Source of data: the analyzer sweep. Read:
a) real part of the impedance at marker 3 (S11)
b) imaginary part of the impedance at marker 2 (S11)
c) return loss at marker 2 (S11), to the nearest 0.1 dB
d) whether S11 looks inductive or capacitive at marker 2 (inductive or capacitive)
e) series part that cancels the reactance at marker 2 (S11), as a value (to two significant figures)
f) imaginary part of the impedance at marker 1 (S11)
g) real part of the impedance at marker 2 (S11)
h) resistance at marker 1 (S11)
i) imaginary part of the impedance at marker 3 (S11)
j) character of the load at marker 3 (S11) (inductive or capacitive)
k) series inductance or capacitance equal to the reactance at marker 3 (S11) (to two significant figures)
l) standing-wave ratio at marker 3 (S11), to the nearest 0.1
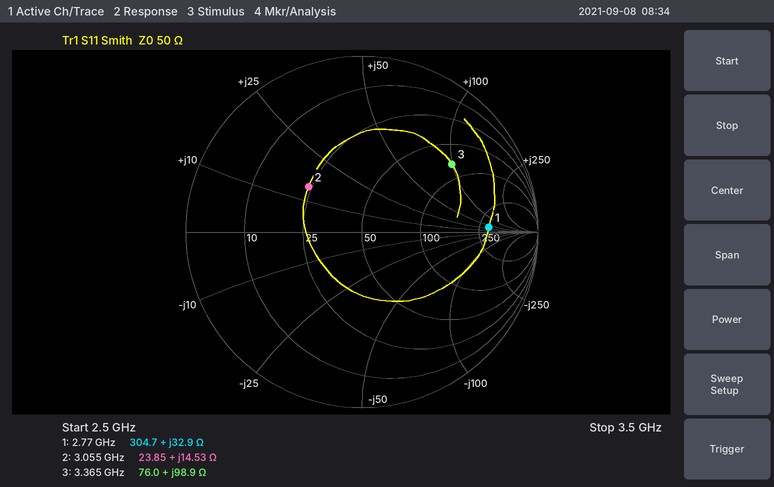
76.0 Ω
+14.53 Ω
8.0 dB
inductive
3.6 pF
+32.9 Ω
23.85 Ω
304.7 Ω
+98.9 Ω
inductive
4.7 nH
4.5
